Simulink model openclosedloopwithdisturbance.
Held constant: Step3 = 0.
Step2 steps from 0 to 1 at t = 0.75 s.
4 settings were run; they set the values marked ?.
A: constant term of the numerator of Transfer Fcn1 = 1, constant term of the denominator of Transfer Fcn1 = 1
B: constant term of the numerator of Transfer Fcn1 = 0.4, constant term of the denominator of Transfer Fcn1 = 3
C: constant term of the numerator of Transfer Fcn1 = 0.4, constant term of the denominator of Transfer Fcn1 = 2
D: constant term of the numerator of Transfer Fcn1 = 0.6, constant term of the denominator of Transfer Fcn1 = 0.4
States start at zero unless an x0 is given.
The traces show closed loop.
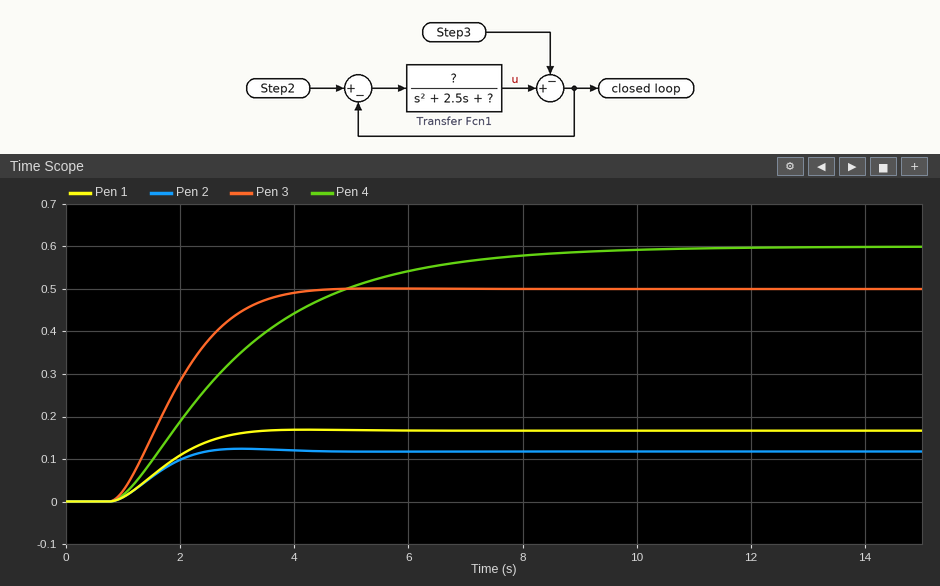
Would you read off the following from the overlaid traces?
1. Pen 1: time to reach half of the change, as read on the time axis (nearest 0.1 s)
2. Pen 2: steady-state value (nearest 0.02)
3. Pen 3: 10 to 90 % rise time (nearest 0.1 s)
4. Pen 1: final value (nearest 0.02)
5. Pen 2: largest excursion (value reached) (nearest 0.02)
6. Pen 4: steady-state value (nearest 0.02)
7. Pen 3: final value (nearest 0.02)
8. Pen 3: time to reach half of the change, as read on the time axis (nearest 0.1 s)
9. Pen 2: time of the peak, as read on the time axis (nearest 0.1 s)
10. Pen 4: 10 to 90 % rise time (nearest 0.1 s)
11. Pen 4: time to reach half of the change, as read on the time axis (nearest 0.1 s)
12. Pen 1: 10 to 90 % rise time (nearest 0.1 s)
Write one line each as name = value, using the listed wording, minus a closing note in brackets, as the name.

Pen 1: time to reach half of the change, as read on the time axis = 1.7 s
Pen 2: steady-state value = 0.12
Pen 3: 10 to 90 % rise time = 2.0 s
Pen 1: final value = 0.16
Pen 2: largest excursion (value reached) = 0.12
Pen 4: steady-state value = 0.60
Pen 3: final value = 0.50
Pen 3: time to reach half of the change, as read on the time axis = 1.9 s
Pen 2: time of the peak, as read on the time axis = 3.1 s
Pen 4: 10 to 90 % rise time = 4.6 s
Pen 4: time to reach half of the change, as read on the time axis = 2.7 s
Pen 1: 10 to 90 % rise time = 1.6 s
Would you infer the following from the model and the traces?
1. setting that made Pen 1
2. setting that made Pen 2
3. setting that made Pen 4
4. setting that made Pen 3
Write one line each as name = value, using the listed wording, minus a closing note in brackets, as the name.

setting that made Pen 1 = C
setting that made Pen 2 = B
setting that made Pen 4 = D
setting that made Pen 3 = A
